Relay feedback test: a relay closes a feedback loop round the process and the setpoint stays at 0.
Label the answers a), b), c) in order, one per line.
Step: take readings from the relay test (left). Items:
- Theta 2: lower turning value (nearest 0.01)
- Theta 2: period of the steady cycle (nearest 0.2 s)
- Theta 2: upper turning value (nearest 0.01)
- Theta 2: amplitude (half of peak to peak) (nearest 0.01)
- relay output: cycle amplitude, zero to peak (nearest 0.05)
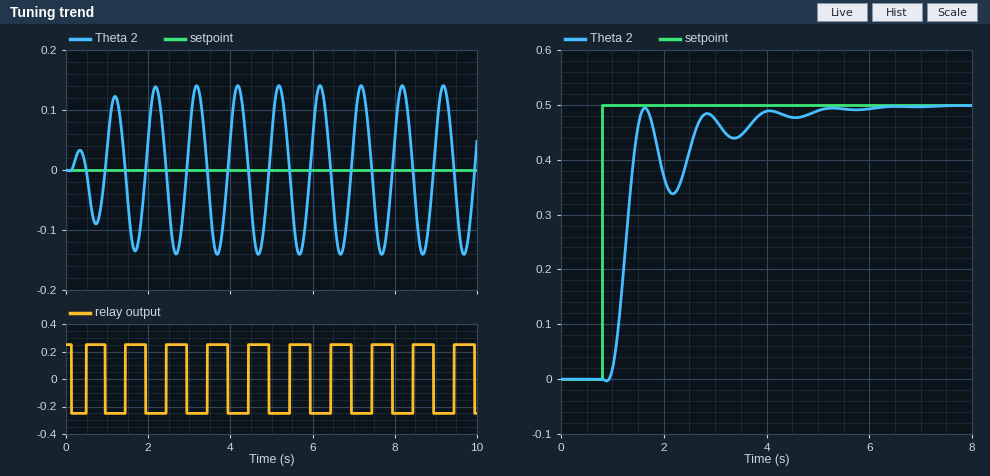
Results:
a) -0.14
b) 1.0 s
c) 0.14
d) 0.14
e) 0.25
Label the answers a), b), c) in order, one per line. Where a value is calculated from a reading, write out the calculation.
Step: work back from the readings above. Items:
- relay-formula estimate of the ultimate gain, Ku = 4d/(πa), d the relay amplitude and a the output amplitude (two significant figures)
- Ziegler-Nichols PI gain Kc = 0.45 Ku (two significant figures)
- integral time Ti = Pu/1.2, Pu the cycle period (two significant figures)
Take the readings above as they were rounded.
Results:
a) 4 × 0.25 / (π × 0.14) = 2.3
b) 0.45 × 2.3 = 1.0
c) 1 / 1.2 = 0.83 s
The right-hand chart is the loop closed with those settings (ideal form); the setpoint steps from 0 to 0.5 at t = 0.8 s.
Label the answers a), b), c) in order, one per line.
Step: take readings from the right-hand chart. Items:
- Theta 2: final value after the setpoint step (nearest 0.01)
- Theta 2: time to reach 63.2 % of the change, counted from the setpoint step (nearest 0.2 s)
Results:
a) 0.50
b) 0.6 s
